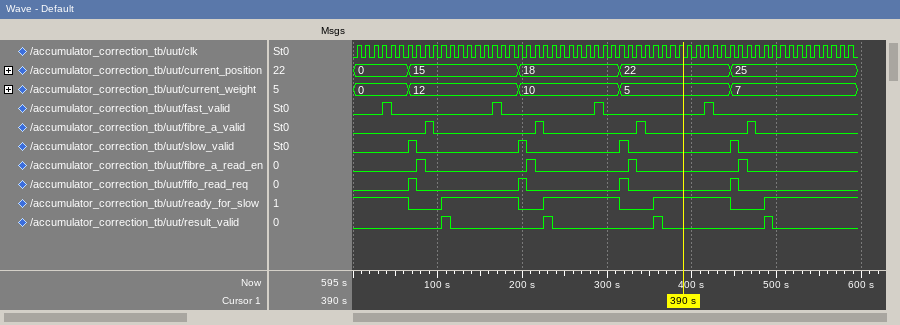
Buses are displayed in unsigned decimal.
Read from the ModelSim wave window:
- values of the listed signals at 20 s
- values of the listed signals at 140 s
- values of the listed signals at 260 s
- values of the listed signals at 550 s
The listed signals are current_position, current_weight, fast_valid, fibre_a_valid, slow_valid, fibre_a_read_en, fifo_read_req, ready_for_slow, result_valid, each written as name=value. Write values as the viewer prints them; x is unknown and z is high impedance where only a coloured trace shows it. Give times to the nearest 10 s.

current_position=0, current_weight=0, fast_valid=0, fibre_a_valid=0, slow_valid=0, fibre_a_read_en=0, fifo_read_req=0, ready_for_slow=1, result_valid=0
current_position=15, current_weight=12, fast_valid=0, fibre_a_valid=0, slow_valid=0, fibre_a_read_en=0, fifo_read_req=0, ready_for_slow=1, result_valid=0
current_position=18, current_weight=10, fast_valid=0, fibre_a_valid=0, slow_valid=0, fibre_a_read_en=0, fifo_read_req=0, ready_for_slow=1, result_valid=0
current_position=25, current_weight=7, fast_valid=0, fibre_a_valid=0, slow_valid=0, fibre_a_read_en=0, fifo_read_req=0, ready_for_slow=1, result_valid=0
